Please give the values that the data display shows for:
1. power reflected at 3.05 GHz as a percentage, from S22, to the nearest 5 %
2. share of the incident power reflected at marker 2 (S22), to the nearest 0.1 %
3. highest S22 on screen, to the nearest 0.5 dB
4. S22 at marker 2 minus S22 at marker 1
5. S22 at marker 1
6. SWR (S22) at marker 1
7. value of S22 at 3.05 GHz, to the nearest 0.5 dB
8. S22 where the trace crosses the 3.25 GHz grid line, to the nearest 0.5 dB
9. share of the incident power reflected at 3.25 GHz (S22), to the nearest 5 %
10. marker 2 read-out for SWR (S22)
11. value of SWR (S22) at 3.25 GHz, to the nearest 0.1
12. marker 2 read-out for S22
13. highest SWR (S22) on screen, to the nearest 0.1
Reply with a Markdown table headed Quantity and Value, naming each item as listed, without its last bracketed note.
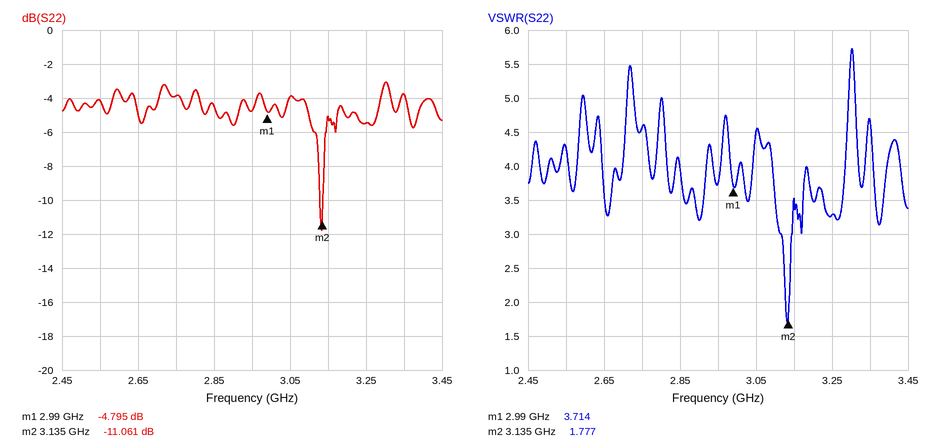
| Quantity | Value |
|---|---|
| power reflected at 3.05 GHz as a percentage, from S22, to the nearest 5 % | 40 % |
| share of the incident power reflected at marker 2 (S22), to the nearest 0.1 % | 7.8 % |
| highest S22 on screen, to the nearest 0.5 dB | -3.0 dB |
| S22 at marker 2 minus S22 at marker 1 | -6.266 dB |
| S22 at marker 1 | -4.795 dB |
| SWR (S22) at marker 1 | 3.714 |
| value of S22 at 3.05 GHz, to the nearest 0.5 dB | -4.0 dB |
| S22 where the trace crosses the 3.25 GHz grid line, to the nearest 0.5 dB | -5.5 dB |
| share of the incident power reflected at 3.25 GHz (S22), to the nearest 5 % | 30 % |
| marker 2 read-out for SWR | 1.777 |
| value of SWR (S22) at 3.25 GHz, to the nearest 0.1 | 3.3 |
| marker 2 read-out for S22 | -11.061 dB |
| highest SWR (S22) on screen, to the nearest 0.1 | 5.7 |
